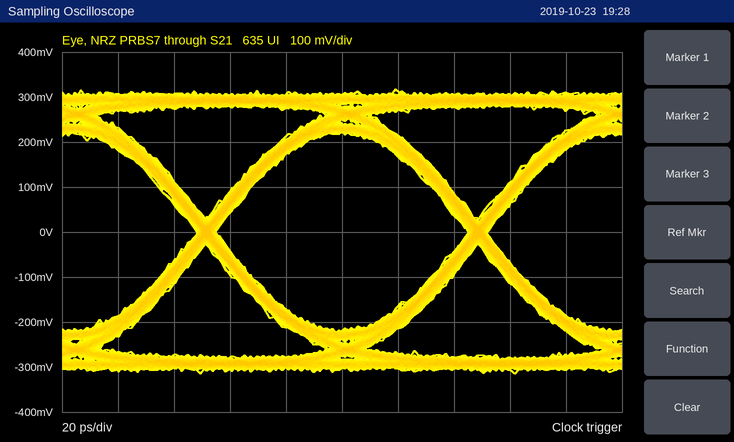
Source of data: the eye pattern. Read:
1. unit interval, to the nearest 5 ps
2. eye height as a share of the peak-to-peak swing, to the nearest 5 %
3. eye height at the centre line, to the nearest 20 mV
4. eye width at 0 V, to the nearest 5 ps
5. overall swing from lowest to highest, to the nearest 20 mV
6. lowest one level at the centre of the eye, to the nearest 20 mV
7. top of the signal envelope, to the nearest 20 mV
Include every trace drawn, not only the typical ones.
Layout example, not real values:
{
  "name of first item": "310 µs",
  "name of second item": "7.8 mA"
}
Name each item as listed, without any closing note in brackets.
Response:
{
  "unit interval, to the nearest 5 ps": "95 ps",
  "eye height as a share of the peak-to-peak swing, to the nearest 5 %": "70 %",
  "eye height at the centre line, to the nearest 20 mV": "440 mV",
  "eye width at 0 V, to the nearest 5 ps": "90 ps",
  "overall swing from lowest to highest, to the nearest 20 mV": "640 mV",
  "lowest one level at the centre of the eye, to the nearest 20 mV": "220 mV",
  "top of the signal envelope, to the nearest 20 mV": "320 mV"
}
